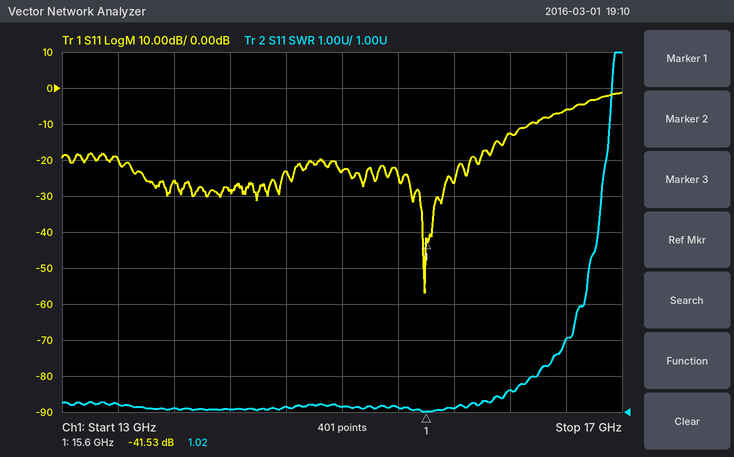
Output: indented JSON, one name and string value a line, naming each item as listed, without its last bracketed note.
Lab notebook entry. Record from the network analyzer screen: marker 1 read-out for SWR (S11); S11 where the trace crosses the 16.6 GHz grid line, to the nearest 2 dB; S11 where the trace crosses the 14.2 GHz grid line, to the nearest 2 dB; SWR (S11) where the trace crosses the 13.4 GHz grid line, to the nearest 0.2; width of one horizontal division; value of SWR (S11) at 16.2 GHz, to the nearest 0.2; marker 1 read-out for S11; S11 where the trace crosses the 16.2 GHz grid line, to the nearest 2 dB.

{
  "marker 1 read-out for SWR": "1.02",
  "S11 where the trace crosses the 16.6 GHz grid line, to the nearest 2 dB": "-6 dB",
  "S11 where the trace crosses the 14.2 GHz grid line, to the nearest 2 dB": "-28 dB",
  "SWR (S11) where the trace crosses the 13.4 GHz grid line, to the nearest 0.2": "1.2",
  "width of one horizontal division": "400 MHz",
  "value of SWR (S11) at 16.2 GHz, to the nearest 0.2": "1.6",
  "marker 1 read-out for S11": "-41.53 dB",
  "S11 where the trace crosses the 16.2 GHz grid line, to the nearest 2 dB": "-12 dB"
}
